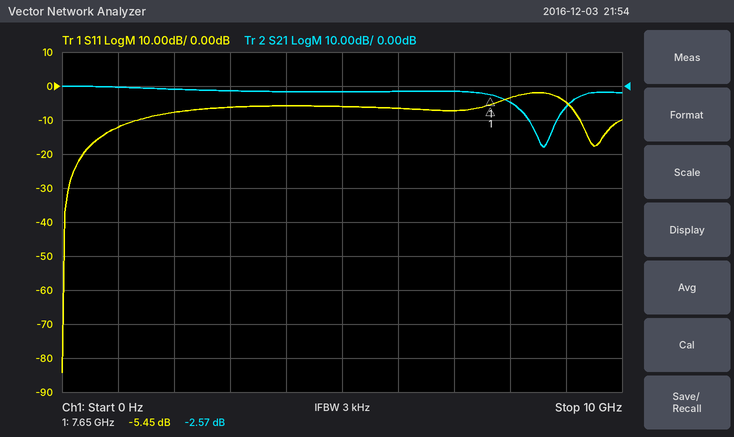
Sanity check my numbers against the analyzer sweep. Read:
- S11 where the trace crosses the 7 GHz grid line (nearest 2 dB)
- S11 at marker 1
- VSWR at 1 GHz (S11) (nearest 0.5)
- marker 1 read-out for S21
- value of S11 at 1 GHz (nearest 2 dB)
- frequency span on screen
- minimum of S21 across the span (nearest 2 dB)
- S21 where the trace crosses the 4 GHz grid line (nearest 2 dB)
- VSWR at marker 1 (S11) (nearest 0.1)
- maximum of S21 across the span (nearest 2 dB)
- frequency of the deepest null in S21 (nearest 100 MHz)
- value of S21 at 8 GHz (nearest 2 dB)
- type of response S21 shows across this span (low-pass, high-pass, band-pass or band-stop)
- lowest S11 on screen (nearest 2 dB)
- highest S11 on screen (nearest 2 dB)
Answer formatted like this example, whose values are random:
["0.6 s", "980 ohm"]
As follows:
["-8 dB", "-5.45 dB", "1.5", "-2.57 dB", "-12 dB", "10 GHz", "-18 dB", "-2 dB", "3.3", "0 dB", "8.6 GHz", "-4 dB", "band-stop", "-84 dB", "-2 dB"]
